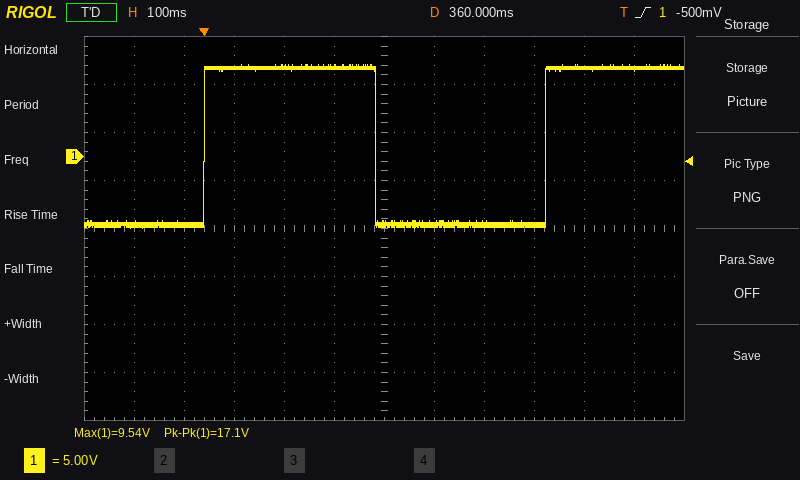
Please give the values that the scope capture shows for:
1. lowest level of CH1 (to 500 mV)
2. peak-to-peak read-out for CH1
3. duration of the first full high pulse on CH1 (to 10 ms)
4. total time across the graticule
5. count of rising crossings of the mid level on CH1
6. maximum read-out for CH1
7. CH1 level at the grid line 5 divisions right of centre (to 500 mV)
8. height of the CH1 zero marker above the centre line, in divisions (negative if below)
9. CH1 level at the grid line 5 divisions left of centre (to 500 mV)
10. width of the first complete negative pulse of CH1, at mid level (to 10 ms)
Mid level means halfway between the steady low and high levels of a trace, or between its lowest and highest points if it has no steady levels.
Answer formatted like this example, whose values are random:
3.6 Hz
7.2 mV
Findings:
-7.5 V
17.1 V
340 ms
1.2 s
2
9.54 V
9.0 V
+1.5 div
-7.0 V
340 ms
